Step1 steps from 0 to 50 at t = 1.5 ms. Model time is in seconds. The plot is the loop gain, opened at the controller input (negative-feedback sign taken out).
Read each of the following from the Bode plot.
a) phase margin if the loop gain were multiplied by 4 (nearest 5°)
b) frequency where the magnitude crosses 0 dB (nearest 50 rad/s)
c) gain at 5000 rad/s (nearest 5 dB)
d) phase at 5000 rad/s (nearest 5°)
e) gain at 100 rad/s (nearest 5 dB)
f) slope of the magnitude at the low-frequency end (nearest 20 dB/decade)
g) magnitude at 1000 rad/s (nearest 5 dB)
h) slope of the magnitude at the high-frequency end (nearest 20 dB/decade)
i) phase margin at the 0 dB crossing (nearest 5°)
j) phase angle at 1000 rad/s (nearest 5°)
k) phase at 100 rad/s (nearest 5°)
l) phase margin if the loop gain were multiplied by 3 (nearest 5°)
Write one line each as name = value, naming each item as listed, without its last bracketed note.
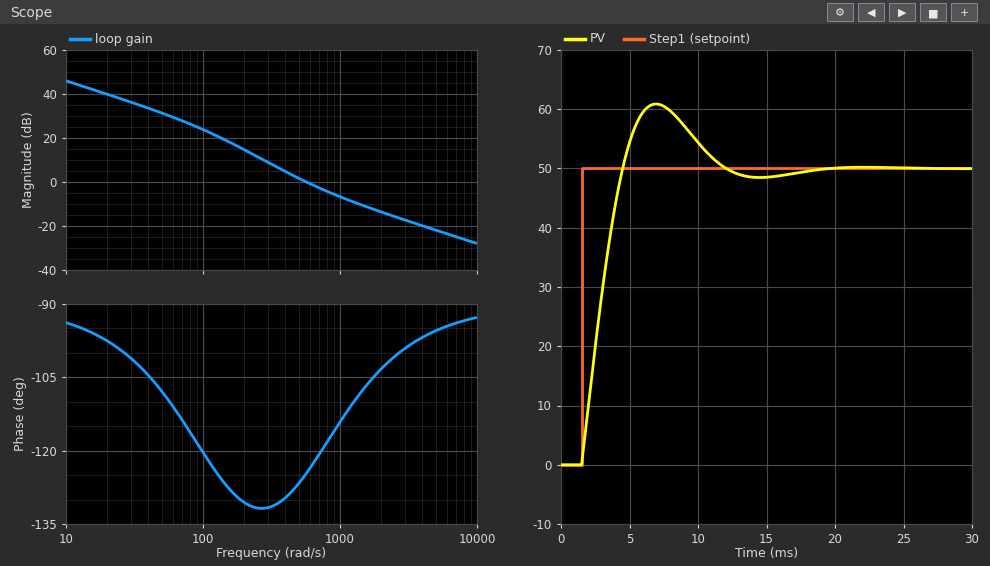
phase margin if the loop gain were multiplied by 4 = 75°
frequency where the magnitude crosses 0 dB = 550 rad/s
gain at 5000 rad/s = -20 dB
phase at 5000 rad/s = -95°
gain at 100 rad/s = 25 dB
slope of the magnitude at the low-frequency end = -20 dB/decade
magnitude at 1000 rad/s = -5 dB
slope of the magnitude at the high-frequency end = -20 dB/decade
phase margin at the 0 dB crossing = 55°
phase angle at 1000 rad/s = -115°
phase at 100 rad/s = -120°
phase margin if the loop gain were multiplied by 3 = 70°
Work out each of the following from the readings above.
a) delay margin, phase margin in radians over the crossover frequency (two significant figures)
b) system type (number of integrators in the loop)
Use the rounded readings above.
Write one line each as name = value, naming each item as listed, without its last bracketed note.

delay margin, phase margin in radians over the crossover frequency = 0.0017 s
system type = 1
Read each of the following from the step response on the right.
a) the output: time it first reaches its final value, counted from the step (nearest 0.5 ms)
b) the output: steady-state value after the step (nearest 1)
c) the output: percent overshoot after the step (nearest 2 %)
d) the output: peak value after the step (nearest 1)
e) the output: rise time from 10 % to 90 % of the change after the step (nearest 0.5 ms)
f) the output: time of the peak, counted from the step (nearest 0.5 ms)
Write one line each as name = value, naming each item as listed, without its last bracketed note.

the output: time it first reaches its final value, counted from the step = 3.0 ms
the output: steady-state value after the step = 50
the output: percent overshoot after the step = 22 %
the output: peak value after the step = 61
the output: rise time from 10 % to 90 % of the change after the step = 2.5 ms
the output: time of the peak, counted from the step = 5.5 ms
